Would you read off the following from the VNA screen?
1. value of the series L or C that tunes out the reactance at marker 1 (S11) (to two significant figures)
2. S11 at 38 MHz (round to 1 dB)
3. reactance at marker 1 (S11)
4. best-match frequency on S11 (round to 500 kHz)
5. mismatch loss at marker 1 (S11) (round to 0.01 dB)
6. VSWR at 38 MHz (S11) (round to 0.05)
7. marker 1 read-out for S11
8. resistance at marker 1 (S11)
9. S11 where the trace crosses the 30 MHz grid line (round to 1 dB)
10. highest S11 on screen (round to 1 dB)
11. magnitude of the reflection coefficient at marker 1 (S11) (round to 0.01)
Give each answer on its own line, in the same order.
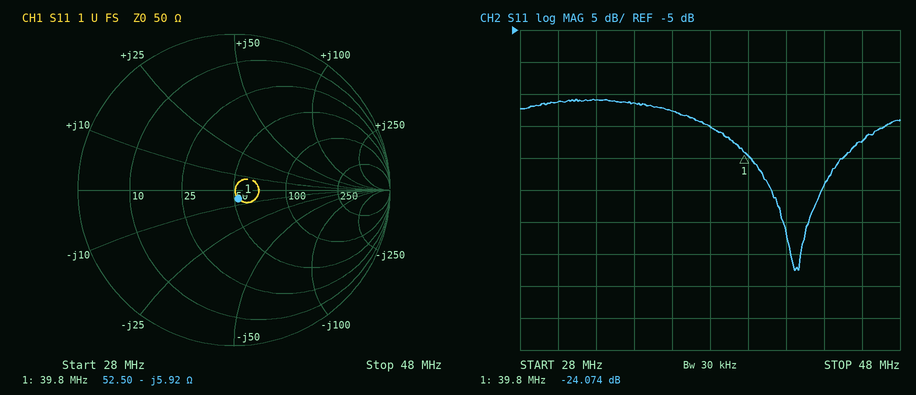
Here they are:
24 nH
-20 dB
-5.92 Ω
42.5 MHz
0.02 dB
1.20
-24.074 dB
52.50 Ω
-16 dB
-16 dB
0.06
